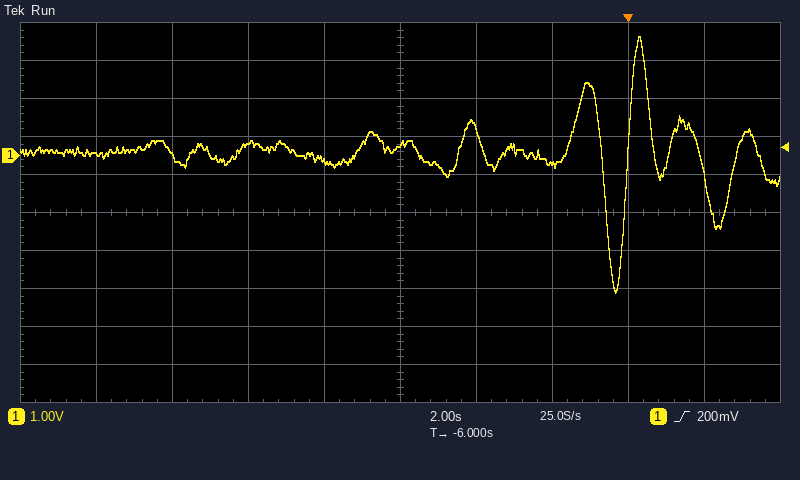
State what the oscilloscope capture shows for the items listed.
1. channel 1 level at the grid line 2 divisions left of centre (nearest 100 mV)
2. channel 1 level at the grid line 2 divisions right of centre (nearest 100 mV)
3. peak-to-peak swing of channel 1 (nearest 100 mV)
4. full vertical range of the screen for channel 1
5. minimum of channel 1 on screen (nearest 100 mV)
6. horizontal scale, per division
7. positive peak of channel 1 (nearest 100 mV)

300 mV
-200 mV
6.7 V
10 V
-3.6 V
2 s
3.1 V
